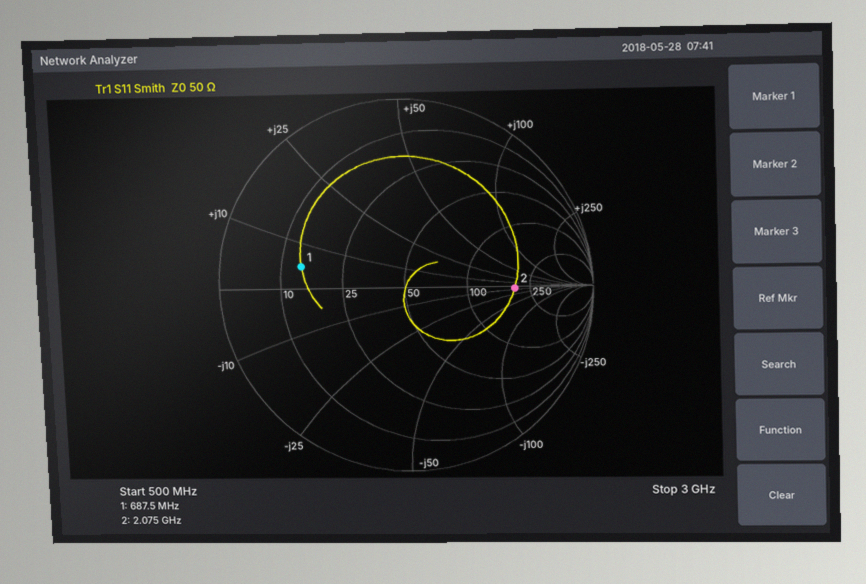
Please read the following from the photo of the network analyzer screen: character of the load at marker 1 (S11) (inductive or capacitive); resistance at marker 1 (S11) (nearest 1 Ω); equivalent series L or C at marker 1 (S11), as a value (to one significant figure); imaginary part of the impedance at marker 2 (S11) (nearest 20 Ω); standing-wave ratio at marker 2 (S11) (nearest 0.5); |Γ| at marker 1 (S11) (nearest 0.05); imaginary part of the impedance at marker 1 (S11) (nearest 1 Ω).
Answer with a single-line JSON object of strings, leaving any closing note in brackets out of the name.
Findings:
{"character of the load at marker 1 (S11)": "inductive", "resistance at marker 1 (S11)": "14 Ω", "equivalent series L or C at marker 1 (S11), as a value": "1 nH", "imaginary part of the impedance at marker 2 (S11)": "0 Ω", "standing-wave ratio at marker 2 (S11)": "4.0", "|Γ| at marker 1 (S11)": "0.55", "imaginary part of the impedance at marker 1 (S11)": "+5 Ω"}
